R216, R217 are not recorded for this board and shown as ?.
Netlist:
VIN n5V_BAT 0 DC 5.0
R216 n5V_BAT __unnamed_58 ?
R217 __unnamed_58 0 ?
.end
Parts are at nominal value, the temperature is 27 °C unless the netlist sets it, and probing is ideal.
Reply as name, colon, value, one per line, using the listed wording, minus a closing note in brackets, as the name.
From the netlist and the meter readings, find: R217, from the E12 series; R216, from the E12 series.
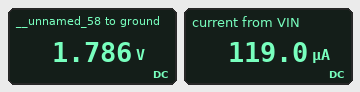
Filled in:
R217, from the E12 series: 15 kΩ
R216, from the E12 series: 27 kΩ
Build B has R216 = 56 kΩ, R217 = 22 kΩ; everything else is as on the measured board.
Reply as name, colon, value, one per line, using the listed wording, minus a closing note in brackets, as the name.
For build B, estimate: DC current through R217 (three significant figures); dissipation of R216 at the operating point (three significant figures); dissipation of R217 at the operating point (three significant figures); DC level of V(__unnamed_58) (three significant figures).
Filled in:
DC current through R217: 64.1 µA
dissipation of R216 at the operating point: 230 µW
dissipation of R217 at the operating point: 90.4 µW
DC level of V(__unnamed_58): 1.41 V
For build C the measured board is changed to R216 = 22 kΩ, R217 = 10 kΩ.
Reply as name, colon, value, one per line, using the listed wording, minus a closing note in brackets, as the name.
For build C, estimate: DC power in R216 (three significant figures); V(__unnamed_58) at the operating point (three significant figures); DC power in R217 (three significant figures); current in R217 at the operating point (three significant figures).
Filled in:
DC power in R216: 537 µW
V(__unnamed_58) at the operating point: 1.56 V
DC power in R217: 244 µW
current in R217 at the operating point: 156 µA
